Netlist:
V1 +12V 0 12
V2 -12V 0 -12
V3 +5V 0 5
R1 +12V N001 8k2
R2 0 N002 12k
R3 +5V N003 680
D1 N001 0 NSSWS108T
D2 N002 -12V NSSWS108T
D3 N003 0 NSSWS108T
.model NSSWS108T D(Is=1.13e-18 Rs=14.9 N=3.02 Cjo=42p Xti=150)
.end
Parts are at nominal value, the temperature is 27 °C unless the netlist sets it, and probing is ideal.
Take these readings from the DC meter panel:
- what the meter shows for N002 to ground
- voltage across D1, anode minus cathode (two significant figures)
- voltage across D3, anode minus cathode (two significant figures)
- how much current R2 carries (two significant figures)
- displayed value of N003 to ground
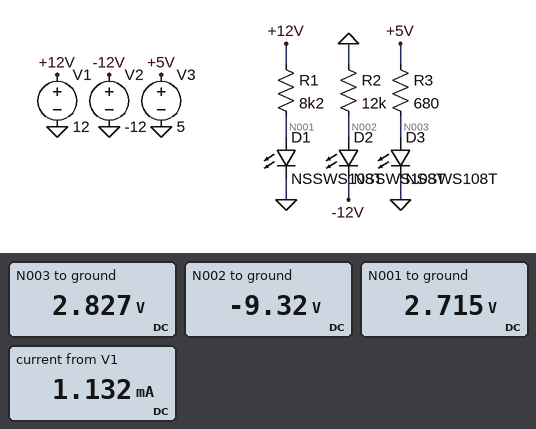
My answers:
-9.32 V
2.7 V
2.8 V
780 µA
2.827 V
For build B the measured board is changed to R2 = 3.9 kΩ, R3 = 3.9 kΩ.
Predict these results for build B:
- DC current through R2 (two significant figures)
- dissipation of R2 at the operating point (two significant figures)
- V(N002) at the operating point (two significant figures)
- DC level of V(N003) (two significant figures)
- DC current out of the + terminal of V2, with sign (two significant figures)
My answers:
2.4 mA
22 mW
-9.2 V
2.7 V
-2.4 mA
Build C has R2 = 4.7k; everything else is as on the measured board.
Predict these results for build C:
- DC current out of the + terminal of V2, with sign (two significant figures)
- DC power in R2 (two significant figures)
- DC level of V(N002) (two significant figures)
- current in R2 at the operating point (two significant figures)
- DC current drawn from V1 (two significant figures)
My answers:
-2.0 mA
18 mW
-9.2 V
2.0 mA
1.1 mA
